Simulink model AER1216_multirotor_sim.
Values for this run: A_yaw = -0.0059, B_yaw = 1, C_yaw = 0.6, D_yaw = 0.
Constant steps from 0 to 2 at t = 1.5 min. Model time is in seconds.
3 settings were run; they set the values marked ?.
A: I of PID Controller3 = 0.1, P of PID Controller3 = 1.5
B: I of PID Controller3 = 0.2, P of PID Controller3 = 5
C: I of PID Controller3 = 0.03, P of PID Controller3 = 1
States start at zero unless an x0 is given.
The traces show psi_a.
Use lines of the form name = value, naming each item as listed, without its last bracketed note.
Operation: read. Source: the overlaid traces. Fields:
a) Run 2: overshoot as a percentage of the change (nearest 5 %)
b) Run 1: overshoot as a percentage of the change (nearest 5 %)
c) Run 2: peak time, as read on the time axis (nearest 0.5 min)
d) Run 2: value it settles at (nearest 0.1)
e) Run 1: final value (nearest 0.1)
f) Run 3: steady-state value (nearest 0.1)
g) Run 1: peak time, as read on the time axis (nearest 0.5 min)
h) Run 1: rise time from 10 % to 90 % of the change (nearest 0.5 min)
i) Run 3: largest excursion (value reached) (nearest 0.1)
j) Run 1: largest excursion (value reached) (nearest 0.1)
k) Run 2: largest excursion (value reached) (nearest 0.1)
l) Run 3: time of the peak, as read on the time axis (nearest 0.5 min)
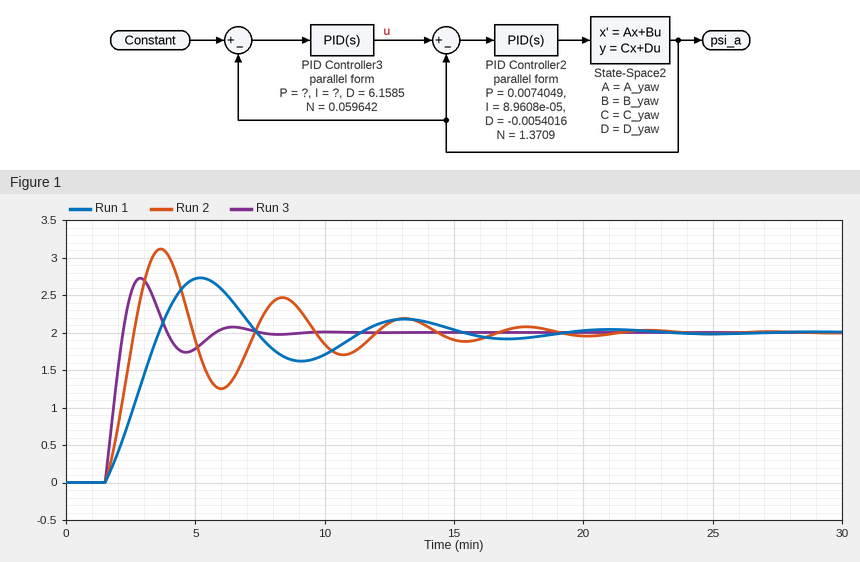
Run 2: overshoot as a percentage of the change = 55 %
Run 1: overshoot as a percentage of the change = 35 %
Run 2: peak time, as read on the time axis = 3.5 min
Run 2: value it settles at = 2.0
Run 1: final value = 2.0
Run 3: steady-state value = 2.0
Run 1: peak time, as read on the time axis = 5.0 min
Run 1: rise time from 10 % to 90 % of the change = 1.5 min
Run 3: largest excursion (value reached) = 2.7
Run 1: largest excursion (value reached) = 2.7
Run 2: largest excursion (value reached) = 3.1
Run 3: time of the peak, as read on the time axis = 3.0 min
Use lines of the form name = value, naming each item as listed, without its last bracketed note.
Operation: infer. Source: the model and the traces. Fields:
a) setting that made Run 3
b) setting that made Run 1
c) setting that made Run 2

setting that made Run 3 = B
setting that made Run 1 = C
setting that made Run 2 = A
